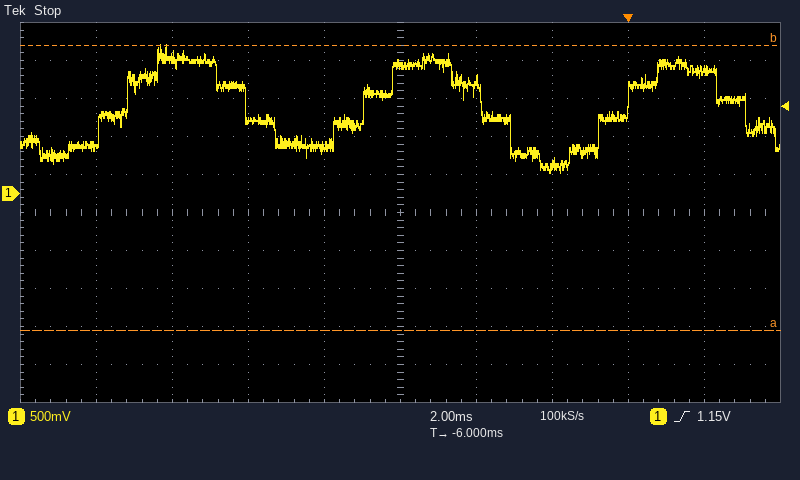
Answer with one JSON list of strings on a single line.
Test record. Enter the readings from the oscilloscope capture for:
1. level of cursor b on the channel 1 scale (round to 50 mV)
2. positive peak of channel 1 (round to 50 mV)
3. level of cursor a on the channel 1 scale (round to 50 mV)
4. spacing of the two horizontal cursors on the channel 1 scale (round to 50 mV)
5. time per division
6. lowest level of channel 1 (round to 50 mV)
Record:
["1.95 V", "1.95 V", "-1.80 V", "3.75 V", "2 ms", "300 mV"]
